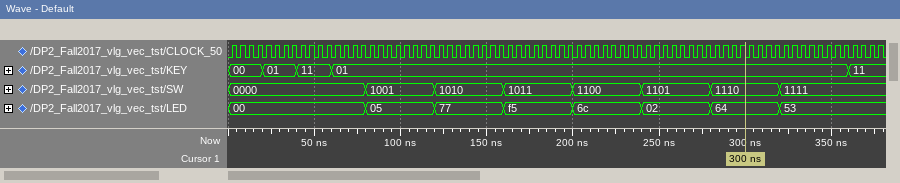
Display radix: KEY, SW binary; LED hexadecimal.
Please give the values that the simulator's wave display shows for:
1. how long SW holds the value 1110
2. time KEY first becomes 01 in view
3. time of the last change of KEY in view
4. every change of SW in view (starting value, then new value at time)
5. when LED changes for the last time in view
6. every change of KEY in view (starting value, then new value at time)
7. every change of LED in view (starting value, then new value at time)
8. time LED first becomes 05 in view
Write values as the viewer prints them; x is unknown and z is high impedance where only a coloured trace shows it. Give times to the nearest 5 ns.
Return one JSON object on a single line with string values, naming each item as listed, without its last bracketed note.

{"how long SW holds the value 1110": "40 ns", "time KEY first becomes 01 in view": "20 ns", "time of the last change of KEY in view": "360 ns", "every change of SW in view": "0000, 1001 at 80 ns, 1010 at 120 ns, 1011 at 160 ns, 1100 at 200 ns, 1101 at 240 ns, 1110 at 280 ns, 1111 at 320 ns", "when LED changes for the last time in view": "320 ns", "every change of KEY in view": "00, 01 at 20 ns, 11 at 40 ns, 01 at 60 ns, 11 at 360 ns", "every change of LED in view": "00, 05 at 80 ns, 77 at 120 ns, f5 at 160 ns, 6c at 200 ns, 02 at 240 ns, 64 at 280 ns, 53 at 320 ns", "time LED first becomes 05 in view": "80 ns"}
